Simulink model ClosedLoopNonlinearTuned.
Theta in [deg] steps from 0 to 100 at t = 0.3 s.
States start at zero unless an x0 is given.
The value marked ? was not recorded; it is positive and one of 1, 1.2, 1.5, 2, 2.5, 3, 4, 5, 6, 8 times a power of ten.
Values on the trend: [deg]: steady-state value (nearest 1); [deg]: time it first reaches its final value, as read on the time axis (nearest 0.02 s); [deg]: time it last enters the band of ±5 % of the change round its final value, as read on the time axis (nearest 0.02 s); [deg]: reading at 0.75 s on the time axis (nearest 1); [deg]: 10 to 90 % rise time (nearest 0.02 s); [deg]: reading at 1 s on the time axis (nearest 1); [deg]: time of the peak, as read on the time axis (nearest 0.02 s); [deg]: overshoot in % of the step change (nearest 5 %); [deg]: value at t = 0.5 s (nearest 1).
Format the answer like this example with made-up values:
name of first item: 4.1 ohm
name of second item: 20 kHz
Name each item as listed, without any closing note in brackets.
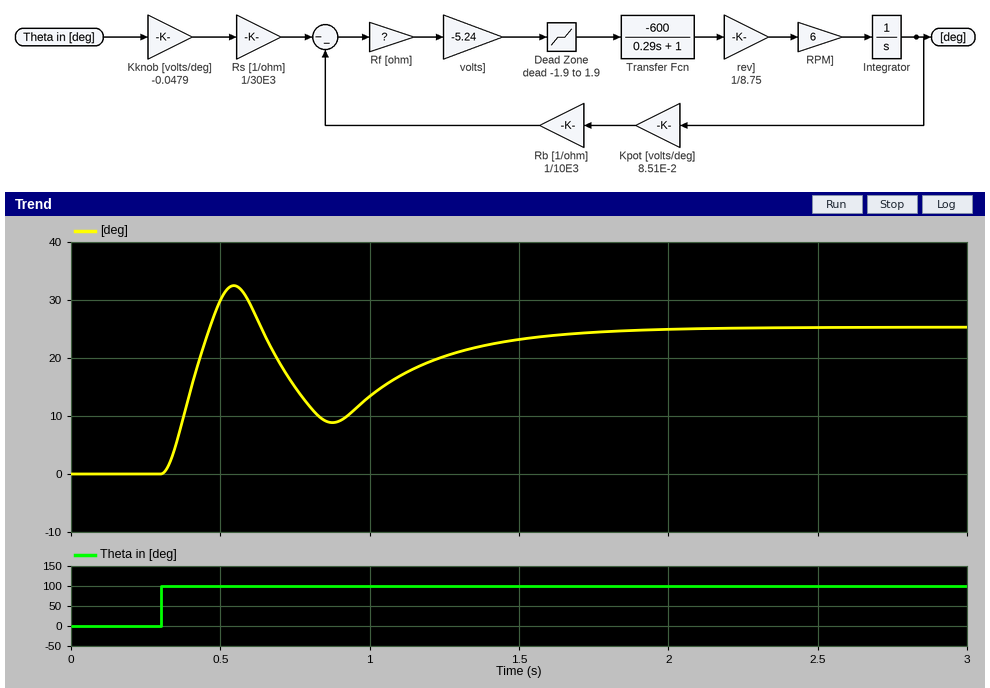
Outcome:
[deg]: steady-state value: 25
[deg]: time it first reaches its final value, as read on the time axis: 0.46 s
[deg]: time it last enters the band of ±5 % of the change round its final value, as read on the time axis: 1.66 s
[deg]: reading at 0.75 s on the time axis: 15
[deg]: 10 to 90 % rise time: 0.12 s
[deg]: reading at 1 s on the time axis: 13
[deg]: time of the peak, as read on the time axis: 0.54 s
[deg]: overshoot in % of the step change: 30 %
[deg]: value at t = 0.5 s: 30
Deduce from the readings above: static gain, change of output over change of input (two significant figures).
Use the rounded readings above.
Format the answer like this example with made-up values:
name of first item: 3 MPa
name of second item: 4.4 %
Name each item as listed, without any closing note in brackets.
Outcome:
static gain, change of output over change of input: 0.25
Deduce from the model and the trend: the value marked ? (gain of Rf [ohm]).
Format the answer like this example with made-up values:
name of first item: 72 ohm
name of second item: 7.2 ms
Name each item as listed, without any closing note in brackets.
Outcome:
the value marked ?: 6000
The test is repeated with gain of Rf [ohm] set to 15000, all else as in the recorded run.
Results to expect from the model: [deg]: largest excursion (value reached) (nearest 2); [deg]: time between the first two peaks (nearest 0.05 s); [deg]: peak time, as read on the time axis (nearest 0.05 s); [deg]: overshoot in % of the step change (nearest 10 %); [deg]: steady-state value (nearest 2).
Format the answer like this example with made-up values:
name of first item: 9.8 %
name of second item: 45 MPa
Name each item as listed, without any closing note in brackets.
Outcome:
[deg]: largest excursion (value reached): 34
[deg]: time between the first two peaks: 0.25 s
[deg]: peak time, as read on the time axis: 0.40 s
[deg]: overshoot in % of the step change: 90 %
[deg]: steady-state value: 18
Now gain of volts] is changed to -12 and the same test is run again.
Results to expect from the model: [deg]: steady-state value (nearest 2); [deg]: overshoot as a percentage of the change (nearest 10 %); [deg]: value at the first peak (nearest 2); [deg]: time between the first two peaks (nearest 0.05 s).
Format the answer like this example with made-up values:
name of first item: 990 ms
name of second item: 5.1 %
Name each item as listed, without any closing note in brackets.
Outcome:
[deg]: steady-state value: 20
[deg]: overshoot as a percentage of the change: 70 %
[deg]: value at the first peak: 34
[deg]: time between the first two peaks: 0.25 s
